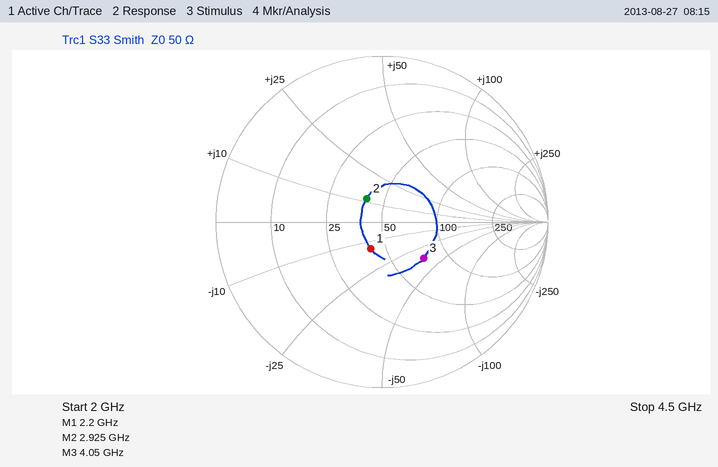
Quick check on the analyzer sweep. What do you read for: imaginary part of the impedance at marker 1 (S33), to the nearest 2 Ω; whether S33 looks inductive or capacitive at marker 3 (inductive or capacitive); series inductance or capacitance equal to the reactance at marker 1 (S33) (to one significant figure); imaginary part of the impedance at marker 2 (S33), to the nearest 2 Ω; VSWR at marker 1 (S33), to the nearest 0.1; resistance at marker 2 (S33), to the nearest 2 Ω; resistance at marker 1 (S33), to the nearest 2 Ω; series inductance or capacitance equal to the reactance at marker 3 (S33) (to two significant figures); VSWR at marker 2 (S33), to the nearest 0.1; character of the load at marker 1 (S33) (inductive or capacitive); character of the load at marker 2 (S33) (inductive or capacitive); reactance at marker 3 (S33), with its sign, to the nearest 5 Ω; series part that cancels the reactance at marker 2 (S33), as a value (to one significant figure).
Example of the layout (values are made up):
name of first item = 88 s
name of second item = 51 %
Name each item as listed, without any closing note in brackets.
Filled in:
imaginary part of the impedance at marker 1 (S33), to the nearest 2 Ω = -14 Ω
whether S33 looks inductive or capacitive at marker 3 = capacitive
series inductance or capacitance equal to the reactance at marker 1 (S33) = 5 pF
imaginary part of the impedance at marker 2 (S33), to the nearest 2 Ω = +12 Ω
VSWR at marker 1 (S33), to the nearest 0.1 = 1.4
resistance at marker 2 (S33), to the nearest 2 Ω = 40 Ω
resistance at marker 1 (S33), to the nearest 2 Ω = 42 Ω
series inductance or capacitance equal to the reactance at marker 3 (S33) = 1.1 pF
VSWR at marker 2 (S33), to the nearest 0.1 = 1.4
character of the load at marker 1 (S33) = capacitive
character of the load at marker 2 (S33) = inductive
reactance at marker 3 (S33), with its sign, to the nearest 5 Ω = -35 Ω
series part that cancels the reactance at marker 2 (S33), as a value = 5 pF
